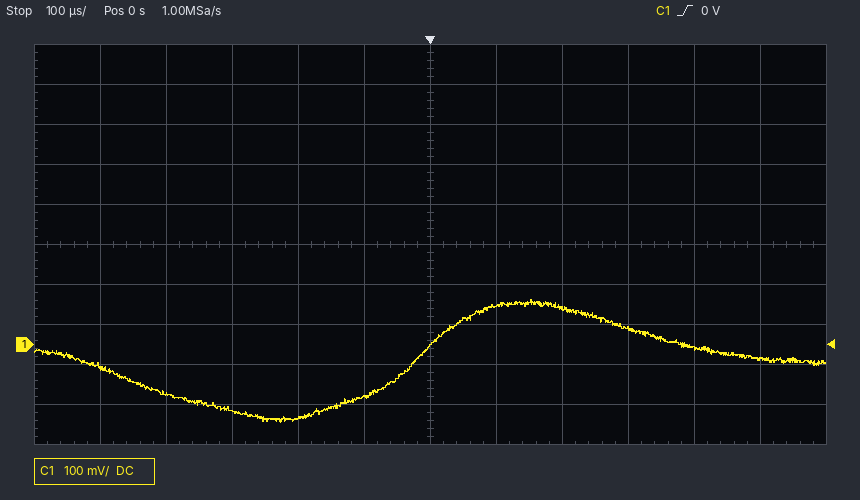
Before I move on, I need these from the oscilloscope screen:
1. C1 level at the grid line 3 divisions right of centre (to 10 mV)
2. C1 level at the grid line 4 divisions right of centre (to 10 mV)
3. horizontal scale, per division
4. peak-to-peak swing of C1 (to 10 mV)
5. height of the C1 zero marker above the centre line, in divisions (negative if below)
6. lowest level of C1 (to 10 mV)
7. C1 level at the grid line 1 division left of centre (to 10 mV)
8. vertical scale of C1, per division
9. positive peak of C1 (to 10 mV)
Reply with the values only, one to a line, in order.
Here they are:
40 mV
-10 mV
100 µs
310 mV
-2.5 div
-200 mV
-130 mV
100 mV
110 mV
